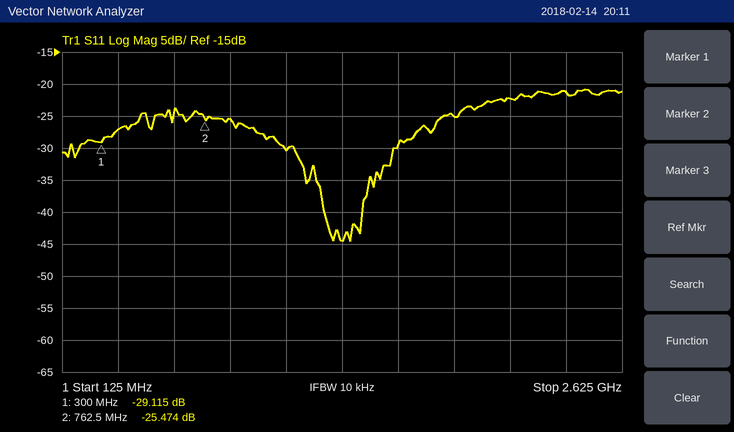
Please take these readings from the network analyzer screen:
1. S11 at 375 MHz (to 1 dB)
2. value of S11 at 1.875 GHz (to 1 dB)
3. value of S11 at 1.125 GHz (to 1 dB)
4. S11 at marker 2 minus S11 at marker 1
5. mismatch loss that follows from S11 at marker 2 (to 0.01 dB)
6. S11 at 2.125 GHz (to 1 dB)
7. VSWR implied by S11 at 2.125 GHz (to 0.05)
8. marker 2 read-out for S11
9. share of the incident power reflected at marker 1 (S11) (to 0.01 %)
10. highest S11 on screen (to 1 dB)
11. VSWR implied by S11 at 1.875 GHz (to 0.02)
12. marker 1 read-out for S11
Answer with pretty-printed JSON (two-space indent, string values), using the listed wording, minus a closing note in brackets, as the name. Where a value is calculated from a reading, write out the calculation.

{
  "S11 at 375 MHz": "-27 dB",
  "value of S11 at 1.875 GHz": "-25 dB",
  "value of S11 at 1.125 GHz": "-30 dB",
  "S11 at marker 2 minus S11 at marker 1": "-25.474 − (-29.115) = 3.641 dB",
  "mismatch loss that follows from S11 at marker 2": "−10 log10(1 − 10^(-25.474/10)) ≈ 0.01 dB",
  "S11 at 2.125 GHz": "-22 dB",
  "VSWR implied by S11 at 2.125 GHz": "|Γ| = 10^(-22/20) = 0.0794; VSWR = (1 + 0.0794)/(1 − 0.0794) ≈ 1.17, so 1.15 to the nearest 0.05",
  "marker 2 read-out for S11": "-25.474 dB",
  "share of the incident power reflected at marker 1 (S11)": "10^(-29.115/10) ≈ 0.12 %",
  "highest S11 on screen": "-21 dB",
  "VSWR implied by S11 at 1.875 GHz": "|Γ| = 10^(-25/20) = 0.0562; VSWR = (1 + 0.0562)/(1 − 0.0562) ≈ 1.12",
  "marker 1 read-out for S11": "-29.115 dB"
}
